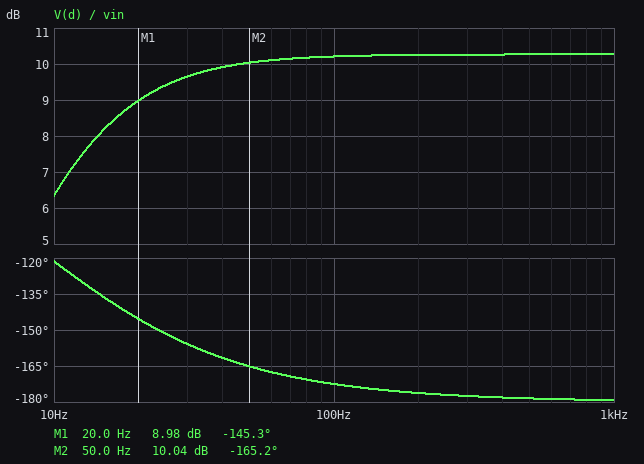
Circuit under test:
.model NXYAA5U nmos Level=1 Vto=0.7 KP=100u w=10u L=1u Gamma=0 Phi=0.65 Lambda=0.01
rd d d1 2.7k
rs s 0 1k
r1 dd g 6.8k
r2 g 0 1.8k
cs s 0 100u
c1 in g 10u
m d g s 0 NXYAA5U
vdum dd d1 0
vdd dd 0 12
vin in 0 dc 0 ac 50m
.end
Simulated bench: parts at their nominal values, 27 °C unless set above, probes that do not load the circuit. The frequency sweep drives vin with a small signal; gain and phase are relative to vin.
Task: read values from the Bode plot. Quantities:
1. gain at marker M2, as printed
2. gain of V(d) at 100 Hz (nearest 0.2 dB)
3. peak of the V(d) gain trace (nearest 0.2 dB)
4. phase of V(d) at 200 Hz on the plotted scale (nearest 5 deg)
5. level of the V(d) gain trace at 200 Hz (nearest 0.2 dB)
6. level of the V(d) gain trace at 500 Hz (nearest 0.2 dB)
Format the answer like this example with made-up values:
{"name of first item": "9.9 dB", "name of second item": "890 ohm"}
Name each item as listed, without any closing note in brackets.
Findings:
{"gain at marker M2, as printed": "10.04 dB", "gain of V(d) at 100 Hz": "10.2 dB", "peak of the V(d) gain trace": "10.2 dB", "phase of V(d) at 200 Hz on the plotted scale": "-175 deg", "level of the V(d) gain trace at 200 Hz": "10.2 dB", "level of the V(d) gain trace at 500 Hz": "10.2 dB"}
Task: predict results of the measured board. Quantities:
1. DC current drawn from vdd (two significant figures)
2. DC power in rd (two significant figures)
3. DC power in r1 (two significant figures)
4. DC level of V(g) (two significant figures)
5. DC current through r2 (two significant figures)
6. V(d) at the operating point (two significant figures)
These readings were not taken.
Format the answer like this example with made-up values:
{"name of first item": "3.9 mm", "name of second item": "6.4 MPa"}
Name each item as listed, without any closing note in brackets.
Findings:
{"DC current drawn from vdd": "2.1 mA", "DC power in rd": "1.3 mW", "DC power in r1": "13 mW", "DC level of V(g)": "2.5 V", "DC current through r2": "1.4 mA", "V(d) at the operating point": "10 V"}
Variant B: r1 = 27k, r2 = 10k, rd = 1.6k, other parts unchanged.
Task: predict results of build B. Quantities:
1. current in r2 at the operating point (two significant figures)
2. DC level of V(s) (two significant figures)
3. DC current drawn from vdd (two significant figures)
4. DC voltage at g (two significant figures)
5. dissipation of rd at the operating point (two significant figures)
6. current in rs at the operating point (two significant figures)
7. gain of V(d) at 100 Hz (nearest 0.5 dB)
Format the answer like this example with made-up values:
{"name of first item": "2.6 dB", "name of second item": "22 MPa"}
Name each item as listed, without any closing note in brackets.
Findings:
{"current in r2 at the operating point": "320 µA", "DC level of V(s)": "1.1 V", "DC current drawn from vdd": "1.4 mA", "DC voltage at g": "3.2 V", "dissipation of rd at the operating point": "2.0 mW", "current in rs at the operating point": "1.1 mA", "gain of V(d) at 100 Hz": "8.0 dB"}
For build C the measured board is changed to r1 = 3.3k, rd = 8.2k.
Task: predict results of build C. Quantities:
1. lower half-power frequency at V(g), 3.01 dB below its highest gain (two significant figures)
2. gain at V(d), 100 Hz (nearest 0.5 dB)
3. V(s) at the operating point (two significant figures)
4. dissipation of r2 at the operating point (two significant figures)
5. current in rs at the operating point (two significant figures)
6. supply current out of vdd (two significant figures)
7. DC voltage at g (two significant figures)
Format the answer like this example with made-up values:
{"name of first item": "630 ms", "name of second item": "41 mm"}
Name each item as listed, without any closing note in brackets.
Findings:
{"lower half-power frequency at V(g), 3.01 dB below its highest gain": "14 Hz", "gain at V(d), 100 Hz": "-9.5 dB", "V(s) at the operating point": "1.2 V", "dissipation of r2 at the operating point": "10 mW", "current in rs at the operating point": "1.2 mA", "supply current out of vdd": "3.6 mA", "DC voltage at g": "4.2 V"}
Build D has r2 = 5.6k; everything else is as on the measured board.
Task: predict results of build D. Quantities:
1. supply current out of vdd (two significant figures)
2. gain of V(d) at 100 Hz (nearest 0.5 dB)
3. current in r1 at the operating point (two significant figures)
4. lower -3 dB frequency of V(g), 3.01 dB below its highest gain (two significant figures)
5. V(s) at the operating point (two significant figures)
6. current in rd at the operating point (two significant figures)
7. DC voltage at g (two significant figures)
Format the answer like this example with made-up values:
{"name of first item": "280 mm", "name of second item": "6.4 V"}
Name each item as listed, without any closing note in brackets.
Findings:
{"supply current out of vdd": "3.5 mA", "gain of V(d) at 100 Hz": "15.0 dB", "current in r1 at the operating point": "970 µA", "lower -3 dB frequency of V(g), 3.01 dB below its highest gain": "5.2 Hz", "V(s) at the operating point": "2.5 V", "current in rd at the operating point": "2.5 mA", "DC voltage at g": "5.4 V"}
